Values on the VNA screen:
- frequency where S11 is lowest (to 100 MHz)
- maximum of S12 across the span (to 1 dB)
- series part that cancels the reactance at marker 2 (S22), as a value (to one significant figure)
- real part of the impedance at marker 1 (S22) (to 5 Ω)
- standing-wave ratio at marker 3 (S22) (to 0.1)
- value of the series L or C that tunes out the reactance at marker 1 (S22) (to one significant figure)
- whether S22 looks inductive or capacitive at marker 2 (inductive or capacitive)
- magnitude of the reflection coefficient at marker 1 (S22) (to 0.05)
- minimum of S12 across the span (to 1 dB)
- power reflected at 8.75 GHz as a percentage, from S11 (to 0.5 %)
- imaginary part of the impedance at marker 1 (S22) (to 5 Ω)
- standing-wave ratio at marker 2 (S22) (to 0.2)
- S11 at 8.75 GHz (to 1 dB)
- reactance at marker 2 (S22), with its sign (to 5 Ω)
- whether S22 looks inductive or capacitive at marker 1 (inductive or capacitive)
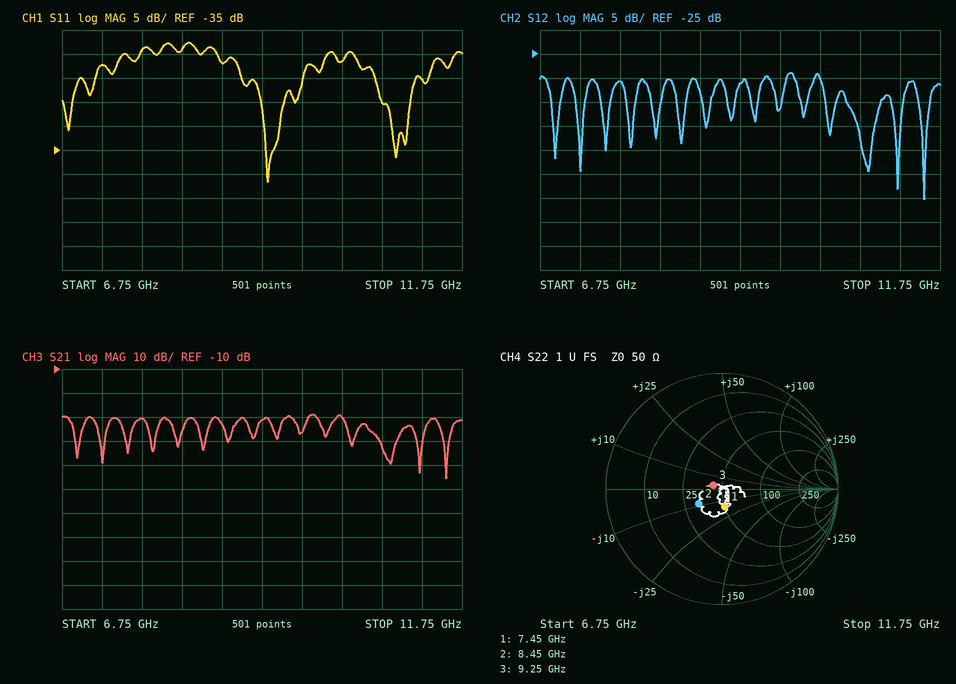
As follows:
9.3 GHz
-29 dB
200 pH
50 Ω
1.2
300 pH
capacitive
0.15
-55 dB
2.0 %
-15 Ω
1.6
-17 dB
-10 Ω
capacitive
